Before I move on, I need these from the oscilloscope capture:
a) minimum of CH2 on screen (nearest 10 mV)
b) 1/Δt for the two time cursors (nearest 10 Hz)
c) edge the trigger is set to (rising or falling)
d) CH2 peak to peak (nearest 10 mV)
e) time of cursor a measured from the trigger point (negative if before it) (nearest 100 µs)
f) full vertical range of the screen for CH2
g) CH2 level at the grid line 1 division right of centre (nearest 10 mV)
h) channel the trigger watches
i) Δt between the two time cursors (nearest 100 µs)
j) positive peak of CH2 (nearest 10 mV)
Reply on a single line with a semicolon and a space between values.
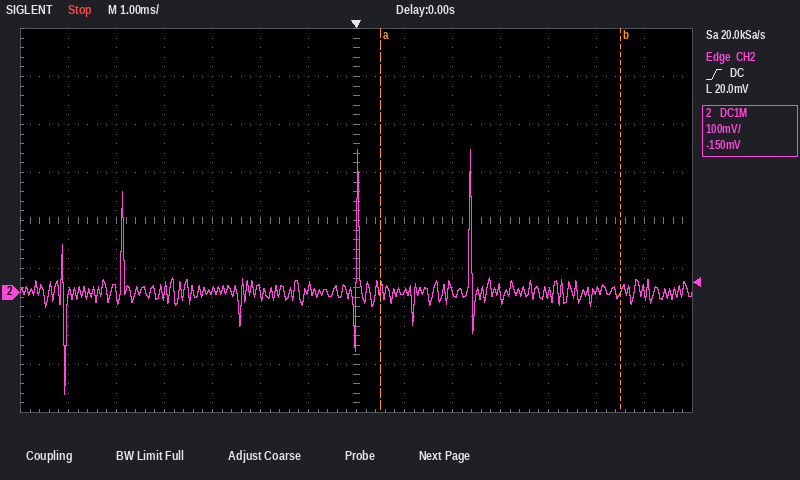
-210 mV; 200 Hz; rising; 510 mV; +500 µs; 800 mV; 0 mV; CH2; 5.0 ms; 300 mV
